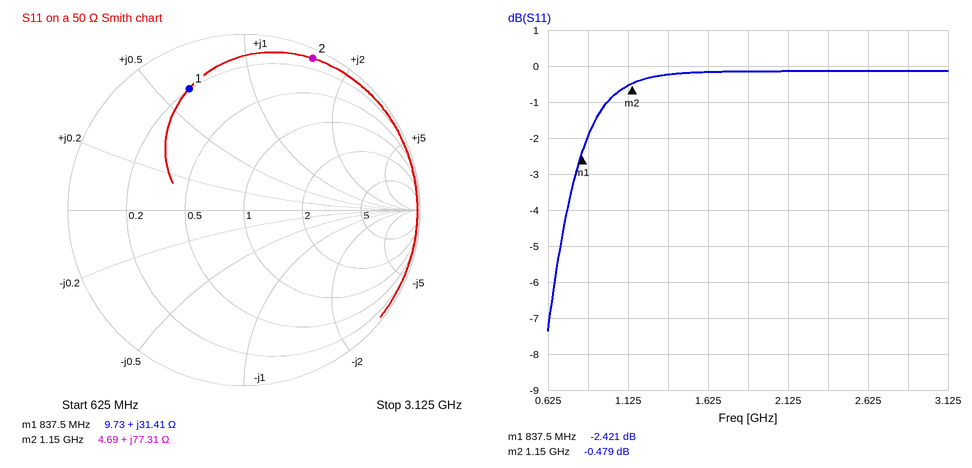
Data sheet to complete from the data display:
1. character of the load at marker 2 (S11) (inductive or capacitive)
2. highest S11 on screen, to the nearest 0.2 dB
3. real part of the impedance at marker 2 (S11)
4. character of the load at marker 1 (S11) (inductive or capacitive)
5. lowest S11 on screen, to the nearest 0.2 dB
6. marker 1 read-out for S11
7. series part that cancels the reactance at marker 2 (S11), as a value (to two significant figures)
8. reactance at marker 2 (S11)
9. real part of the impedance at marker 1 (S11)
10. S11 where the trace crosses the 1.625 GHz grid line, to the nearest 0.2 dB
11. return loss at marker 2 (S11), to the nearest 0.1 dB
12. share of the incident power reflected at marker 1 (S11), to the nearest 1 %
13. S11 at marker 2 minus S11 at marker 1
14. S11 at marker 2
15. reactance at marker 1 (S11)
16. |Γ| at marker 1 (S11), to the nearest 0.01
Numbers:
inductive
-0.2 dB
4.69 Ω
inductive
-7.4 dB
-2.421 dB
1.8 pF
+77.31 Ω
9.73 Ω
-0.2 dB
0.5 dB
57 %
1.942 dB
-0.479 dB
+31.41 Ω
0.76
